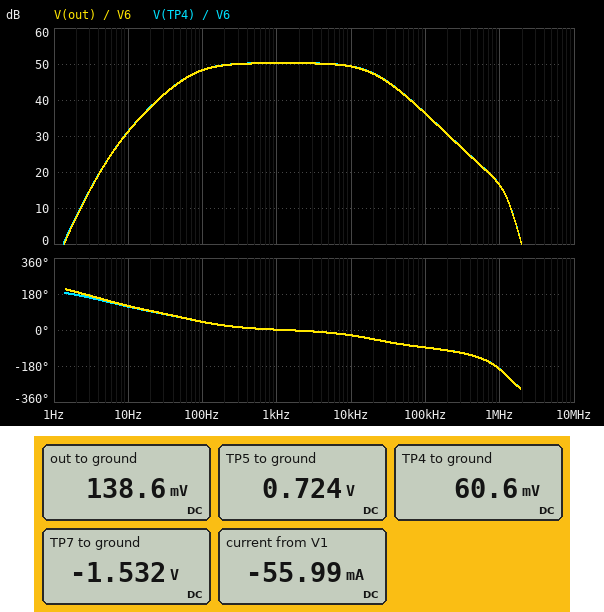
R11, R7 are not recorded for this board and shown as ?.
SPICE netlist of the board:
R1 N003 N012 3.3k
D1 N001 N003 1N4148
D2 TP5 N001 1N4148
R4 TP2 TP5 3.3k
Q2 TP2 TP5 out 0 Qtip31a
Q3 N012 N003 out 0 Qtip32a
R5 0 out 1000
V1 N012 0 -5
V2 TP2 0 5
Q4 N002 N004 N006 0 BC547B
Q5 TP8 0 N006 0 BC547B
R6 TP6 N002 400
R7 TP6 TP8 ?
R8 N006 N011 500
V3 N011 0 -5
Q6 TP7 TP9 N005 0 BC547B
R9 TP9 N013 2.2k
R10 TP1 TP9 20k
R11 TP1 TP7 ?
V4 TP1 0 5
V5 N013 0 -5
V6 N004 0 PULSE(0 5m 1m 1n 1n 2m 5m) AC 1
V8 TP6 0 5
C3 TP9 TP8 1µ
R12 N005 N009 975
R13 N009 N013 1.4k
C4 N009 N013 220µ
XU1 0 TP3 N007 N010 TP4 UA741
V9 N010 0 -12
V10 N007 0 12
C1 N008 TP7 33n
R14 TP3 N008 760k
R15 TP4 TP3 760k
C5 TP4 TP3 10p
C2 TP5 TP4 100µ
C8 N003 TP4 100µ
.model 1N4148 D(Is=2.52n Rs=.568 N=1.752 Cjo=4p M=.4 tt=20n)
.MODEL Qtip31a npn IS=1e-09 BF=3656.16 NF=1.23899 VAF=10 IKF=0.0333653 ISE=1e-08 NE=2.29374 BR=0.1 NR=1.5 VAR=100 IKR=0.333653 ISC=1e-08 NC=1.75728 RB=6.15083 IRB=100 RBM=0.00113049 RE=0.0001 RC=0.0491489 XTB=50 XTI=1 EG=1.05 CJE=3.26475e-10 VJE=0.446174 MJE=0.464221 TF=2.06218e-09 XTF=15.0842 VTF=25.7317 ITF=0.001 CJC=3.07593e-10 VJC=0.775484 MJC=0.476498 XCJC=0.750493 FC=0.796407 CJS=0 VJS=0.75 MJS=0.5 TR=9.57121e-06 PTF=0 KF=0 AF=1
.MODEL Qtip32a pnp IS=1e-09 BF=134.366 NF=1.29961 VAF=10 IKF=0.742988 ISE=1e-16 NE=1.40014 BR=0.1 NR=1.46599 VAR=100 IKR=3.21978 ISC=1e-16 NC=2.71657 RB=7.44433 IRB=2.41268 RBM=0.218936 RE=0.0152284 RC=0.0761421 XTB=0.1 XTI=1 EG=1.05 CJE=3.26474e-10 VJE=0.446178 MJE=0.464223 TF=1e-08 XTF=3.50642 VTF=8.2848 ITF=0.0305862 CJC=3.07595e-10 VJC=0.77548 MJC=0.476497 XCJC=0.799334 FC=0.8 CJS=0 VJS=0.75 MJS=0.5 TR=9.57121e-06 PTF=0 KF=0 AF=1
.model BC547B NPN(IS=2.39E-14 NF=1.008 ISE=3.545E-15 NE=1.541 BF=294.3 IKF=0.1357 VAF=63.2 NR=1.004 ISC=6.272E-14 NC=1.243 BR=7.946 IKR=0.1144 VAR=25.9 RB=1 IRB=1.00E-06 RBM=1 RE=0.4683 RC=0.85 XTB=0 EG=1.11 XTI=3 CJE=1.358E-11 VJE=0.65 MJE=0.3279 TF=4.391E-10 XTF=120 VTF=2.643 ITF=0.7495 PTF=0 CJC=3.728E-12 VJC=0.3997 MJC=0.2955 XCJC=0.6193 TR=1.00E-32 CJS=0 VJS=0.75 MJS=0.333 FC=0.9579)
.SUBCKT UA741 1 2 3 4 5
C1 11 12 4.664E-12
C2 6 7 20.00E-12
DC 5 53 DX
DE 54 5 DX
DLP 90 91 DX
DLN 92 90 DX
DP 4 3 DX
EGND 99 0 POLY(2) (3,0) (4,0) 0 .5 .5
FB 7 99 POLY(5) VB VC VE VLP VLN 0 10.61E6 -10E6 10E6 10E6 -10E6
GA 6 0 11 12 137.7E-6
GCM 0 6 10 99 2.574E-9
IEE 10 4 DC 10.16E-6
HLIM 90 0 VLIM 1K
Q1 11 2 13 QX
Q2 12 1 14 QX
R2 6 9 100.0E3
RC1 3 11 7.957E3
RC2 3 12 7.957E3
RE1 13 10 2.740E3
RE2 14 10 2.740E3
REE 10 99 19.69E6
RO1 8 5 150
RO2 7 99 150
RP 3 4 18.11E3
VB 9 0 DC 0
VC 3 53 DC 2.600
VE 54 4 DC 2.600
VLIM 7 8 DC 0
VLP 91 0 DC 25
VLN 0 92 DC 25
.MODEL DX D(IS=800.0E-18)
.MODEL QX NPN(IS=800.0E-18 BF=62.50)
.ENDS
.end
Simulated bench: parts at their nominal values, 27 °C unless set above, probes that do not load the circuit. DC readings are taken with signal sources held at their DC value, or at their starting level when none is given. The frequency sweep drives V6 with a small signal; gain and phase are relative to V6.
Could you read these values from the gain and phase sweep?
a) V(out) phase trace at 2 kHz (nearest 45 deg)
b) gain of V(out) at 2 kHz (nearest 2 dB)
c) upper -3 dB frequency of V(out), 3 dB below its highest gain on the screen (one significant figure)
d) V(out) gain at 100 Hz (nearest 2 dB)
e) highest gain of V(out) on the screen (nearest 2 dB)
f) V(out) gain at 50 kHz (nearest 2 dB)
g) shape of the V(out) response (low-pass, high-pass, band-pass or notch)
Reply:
0 deg
50 dB
20 kHz
48 dB
50 dB
42 dB
band-pass
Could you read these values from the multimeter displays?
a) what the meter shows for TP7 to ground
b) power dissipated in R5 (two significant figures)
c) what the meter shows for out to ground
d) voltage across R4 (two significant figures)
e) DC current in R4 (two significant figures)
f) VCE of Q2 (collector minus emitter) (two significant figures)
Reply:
-1.532 V
19 µW
138.6 mV
4.3 V
1.3 mA
4.9 V
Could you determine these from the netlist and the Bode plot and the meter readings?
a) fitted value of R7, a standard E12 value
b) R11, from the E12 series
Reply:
150 Ω
39 kΩ
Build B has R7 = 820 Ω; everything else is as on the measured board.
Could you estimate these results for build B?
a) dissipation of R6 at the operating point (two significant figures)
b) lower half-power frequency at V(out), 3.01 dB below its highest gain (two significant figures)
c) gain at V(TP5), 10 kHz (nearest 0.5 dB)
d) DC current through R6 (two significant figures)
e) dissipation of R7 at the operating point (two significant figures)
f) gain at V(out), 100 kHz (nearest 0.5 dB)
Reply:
7.6 mW
58 Hz
61.5 dB
4.4 mA
15 mW
48.5 dB
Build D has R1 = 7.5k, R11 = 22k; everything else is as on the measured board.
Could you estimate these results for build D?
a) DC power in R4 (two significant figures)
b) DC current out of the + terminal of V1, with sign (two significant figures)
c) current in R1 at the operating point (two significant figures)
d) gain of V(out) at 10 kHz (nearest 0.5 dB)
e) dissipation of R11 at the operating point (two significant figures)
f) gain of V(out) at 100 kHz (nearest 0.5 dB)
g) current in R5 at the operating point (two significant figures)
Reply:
2.2 mW
-32 mA
820 µA
44.5 dB
620 µW
31.5 dB
1.7 mA
